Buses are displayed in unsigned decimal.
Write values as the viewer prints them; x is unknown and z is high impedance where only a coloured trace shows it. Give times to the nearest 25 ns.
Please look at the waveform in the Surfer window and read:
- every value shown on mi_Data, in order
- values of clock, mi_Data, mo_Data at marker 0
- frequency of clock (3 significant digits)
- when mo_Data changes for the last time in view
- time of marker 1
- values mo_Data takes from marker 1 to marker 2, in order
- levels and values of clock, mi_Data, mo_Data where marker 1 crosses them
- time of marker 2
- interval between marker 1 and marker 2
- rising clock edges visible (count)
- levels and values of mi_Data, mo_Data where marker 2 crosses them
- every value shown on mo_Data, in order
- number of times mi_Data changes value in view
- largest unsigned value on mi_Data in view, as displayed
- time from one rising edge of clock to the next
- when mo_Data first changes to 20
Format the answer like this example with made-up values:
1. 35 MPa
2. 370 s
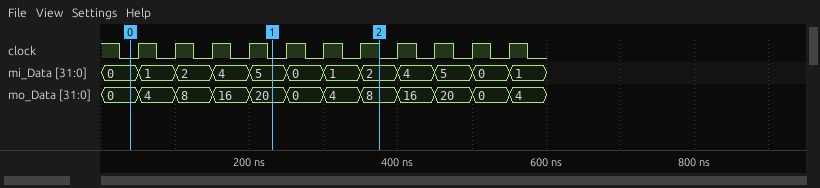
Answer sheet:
1. 0, 1, 2, 4, 5, 0, 1, 2, 4, 5, 0, 1
2. clock=0, mi_Data=0, mo_Data=0
3. 20.0 MHz
4. 550 ns
5. 225 ns
6. 20, 0, 4, 8
7. clock=0, mi_Data=5, mo_Data=20
8. 375 ns
9. 150 ns
10. 11
11. mi_Data=2, mo_Data=8
12. 0, 4, 8, 16, 20, 0, 4, 8, 16, 20, 0, 4
13. 11
14. 5
15. 50 ns
16. 200 ns
